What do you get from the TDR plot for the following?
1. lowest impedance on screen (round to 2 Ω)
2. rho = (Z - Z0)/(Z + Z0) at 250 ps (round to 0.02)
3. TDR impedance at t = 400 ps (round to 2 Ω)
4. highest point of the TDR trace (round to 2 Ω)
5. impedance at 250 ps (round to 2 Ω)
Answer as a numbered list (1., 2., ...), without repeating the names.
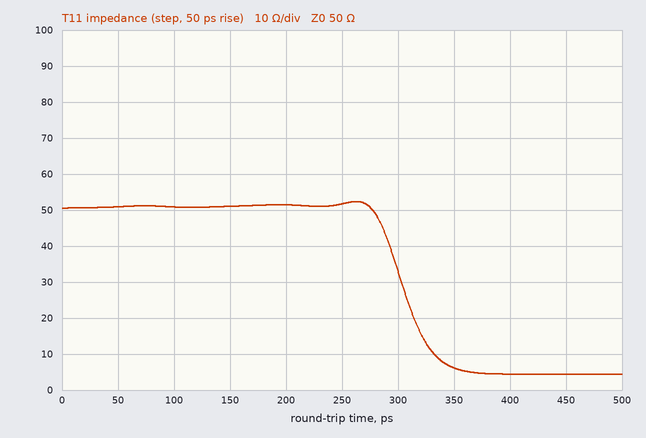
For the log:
1. 4 Ω
2. +0.02
3. 4 Ω
4. 52 Ω
5. 52 Ω
